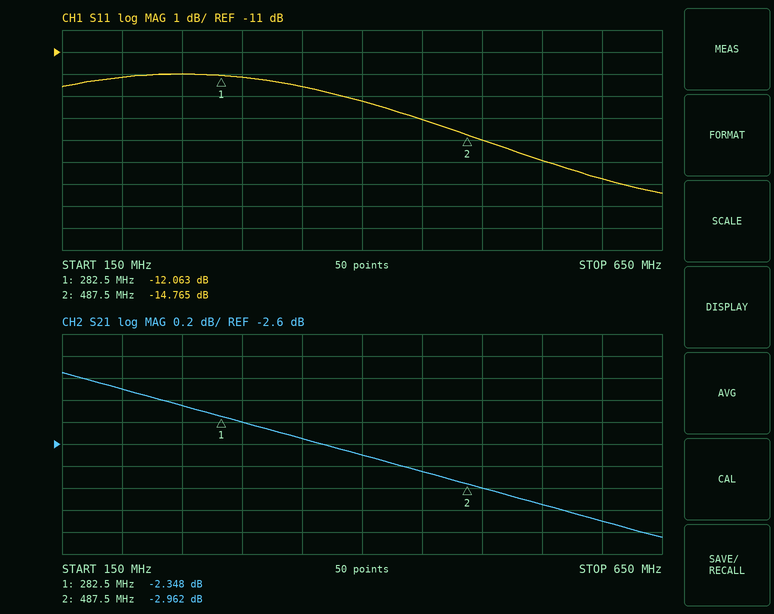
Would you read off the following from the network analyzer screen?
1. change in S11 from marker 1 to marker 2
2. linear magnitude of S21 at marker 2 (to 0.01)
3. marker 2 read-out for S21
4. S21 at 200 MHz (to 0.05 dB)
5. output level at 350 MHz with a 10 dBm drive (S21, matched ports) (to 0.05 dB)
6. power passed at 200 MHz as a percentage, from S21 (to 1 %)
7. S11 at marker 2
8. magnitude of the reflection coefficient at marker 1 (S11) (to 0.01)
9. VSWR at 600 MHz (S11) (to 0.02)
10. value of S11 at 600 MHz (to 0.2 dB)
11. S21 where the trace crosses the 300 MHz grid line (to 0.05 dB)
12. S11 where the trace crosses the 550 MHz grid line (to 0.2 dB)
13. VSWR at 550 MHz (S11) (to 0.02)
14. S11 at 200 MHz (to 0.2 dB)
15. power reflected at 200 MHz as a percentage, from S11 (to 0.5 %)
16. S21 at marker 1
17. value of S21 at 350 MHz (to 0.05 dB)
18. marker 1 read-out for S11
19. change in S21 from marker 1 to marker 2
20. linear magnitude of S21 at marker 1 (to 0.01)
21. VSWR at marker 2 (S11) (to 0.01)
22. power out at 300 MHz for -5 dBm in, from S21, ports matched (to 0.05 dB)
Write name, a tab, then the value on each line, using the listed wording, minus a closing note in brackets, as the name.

change in S11 from marker 1 to marker 2	-2.702 dB
linear magnitude of S21 at marker 2	0.71
marker 2 read-out for S21	-2.962 dB
S21 at 200 MHz	-2.10 dB
output level at 350 MHz with a 10 dBm drive (S21, matched ports)	7.45 dBm
power passed at 200 MHz as a percentage, from S21	62 %
S11 at marker 2	-14.765 dB
magnitude of the reflection coefficient at marker 1 (S11)	0.25
VSWR at 600 MHz (S11)	1.34
value of S11 at 600 MHz	-16.8 dB
S21 where the trace crosses the 300 MHz grid line	-2.40 dB
S11 where the trace crosses the 550 MHz grid line	-16.0 dB
VSWR at 550 MHz (S11)	1.38
S11 at 200 MHz	-12.2 dB
power reflected at 200 MHz as a percentage, from S11	6.0 %
S21 at marker 1	-2.348 dB
value of S21 at 350 MHz	-2.55 dB
marker 1 read-out for S11	-12.063 dB
change in S21 from marker 1 to marker 2	-0.614 dB
linear magnitude of S21 at marker 1	0.76
VSWR at marker 2 (S11)	1.45
power out at 300 MHz for -5 dBm in, from S21, ports matched	-7.40 dBm
